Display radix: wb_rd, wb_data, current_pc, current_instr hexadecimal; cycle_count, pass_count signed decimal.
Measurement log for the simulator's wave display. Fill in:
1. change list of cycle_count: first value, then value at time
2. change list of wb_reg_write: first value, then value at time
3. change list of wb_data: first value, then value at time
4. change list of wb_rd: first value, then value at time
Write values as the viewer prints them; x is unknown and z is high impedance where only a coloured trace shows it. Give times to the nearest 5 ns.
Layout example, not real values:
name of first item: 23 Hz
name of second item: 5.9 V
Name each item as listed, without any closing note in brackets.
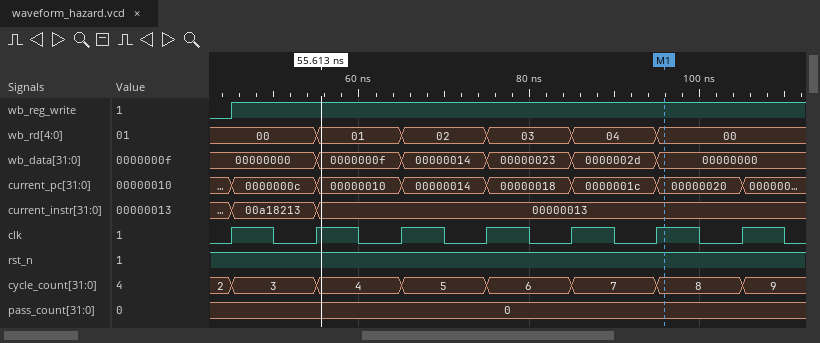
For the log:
change list of cycle_count: first value, then value at time: 2, 3 at 45 ns, 4 at 55 ns, 5 at 65 ns, 6 at 75 ns, 7 at 85 ns, 8 at 95 ns, 9 at 105 ns
change list of wb_reg_write: first value, then value at time: 0, 1 at 45 ns
change list of wb_data: first value, then value at time: 00000000, 0000000f at 55 ns, 00000014 at 65 ns, 00000023 at 75 ns, 0000002d at 85 ns, 00000000 at 95 ns
change list of wb_rd: first value, then value at time: 00, 01 at 55 ns, 02 at 65 ns, 03 at 75 ns, 04 at 85 ns, 00 at 95 ns
